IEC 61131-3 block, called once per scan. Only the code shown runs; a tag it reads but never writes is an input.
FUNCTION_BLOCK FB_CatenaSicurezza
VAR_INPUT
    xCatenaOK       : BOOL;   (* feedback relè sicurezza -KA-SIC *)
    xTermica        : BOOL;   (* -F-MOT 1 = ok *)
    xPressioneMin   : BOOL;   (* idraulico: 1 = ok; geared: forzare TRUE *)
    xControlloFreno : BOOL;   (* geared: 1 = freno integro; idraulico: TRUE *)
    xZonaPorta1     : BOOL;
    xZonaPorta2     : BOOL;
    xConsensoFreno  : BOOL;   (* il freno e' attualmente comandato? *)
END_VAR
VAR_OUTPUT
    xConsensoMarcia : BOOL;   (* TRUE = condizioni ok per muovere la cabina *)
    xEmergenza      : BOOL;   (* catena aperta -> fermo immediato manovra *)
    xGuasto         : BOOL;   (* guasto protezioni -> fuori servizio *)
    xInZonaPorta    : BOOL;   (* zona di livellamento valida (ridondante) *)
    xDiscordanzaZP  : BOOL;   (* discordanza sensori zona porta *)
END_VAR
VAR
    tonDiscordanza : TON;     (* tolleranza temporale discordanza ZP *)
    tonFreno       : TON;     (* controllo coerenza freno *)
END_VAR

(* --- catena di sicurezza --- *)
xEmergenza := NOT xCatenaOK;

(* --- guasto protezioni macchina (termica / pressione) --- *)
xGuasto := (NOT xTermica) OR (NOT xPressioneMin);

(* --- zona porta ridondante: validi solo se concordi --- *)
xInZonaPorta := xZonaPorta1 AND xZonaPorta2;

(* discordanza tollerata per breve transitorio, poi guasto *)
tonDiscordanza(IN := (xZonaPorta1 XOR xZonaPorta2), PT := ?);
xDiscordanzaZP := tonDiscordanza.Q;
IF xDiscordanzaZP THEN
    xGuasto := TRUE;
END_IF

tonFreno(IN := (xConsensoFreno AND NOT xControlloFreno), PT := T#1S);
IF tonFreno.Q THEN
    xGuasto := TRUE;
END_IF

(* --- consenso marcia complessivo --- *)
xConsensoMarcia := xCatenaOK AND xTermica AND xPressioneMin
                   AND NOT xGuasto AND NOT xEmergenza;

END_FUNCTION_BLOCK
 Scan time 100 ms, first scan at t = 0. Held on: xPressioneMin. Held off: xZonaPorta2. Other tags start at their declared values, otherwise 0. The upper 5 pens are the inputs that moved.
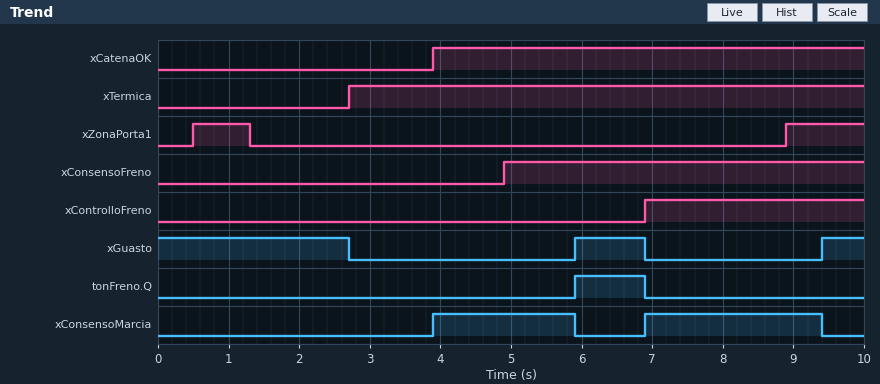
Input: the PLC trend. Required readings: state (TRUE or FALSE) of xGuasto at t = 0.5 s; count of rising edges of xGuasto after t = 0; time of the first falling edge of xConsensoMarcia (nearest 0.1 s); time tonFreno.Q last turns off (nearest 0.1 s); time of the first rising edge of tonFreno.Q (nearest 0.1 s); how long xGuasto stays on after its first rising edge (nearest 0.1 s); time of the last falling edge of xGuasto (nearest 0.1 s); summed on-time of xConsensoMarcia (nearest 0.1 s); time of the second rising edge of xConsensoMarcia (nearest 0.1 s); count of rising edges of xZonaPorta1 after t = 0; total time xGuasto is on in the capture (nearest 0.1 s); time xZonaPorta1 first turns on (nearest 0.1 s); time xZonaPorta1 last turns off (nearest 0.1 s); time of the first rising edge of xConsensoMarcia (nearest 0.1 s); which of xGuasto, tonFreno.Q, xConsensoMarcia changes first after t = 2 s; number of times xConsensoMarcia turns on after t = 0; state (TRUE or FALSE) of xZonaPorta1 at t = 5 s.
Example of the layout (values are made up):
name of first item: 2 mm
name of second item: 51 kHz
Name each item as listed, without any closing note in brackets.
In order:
state (TRUE or FALSE) of xGuasto at t = 0.5 s: TRUE
count of rising edges of xGuasto after t = 0: 2
time of the first falling edge of xConsensoMarcia: 5.9 s
time tonFreno.Q last turns off: 6.9 s
time of the first rising edge of tonFreno.Q: 5.9 s
how long xGuasto stays on after its first rising edge: 1.0 s
time of the last falling edge of xGuasto: 6.9 s
summed on-time of xConsensoMarcia: 4.5 s
time of the second rising edge of xConsensoMarcia: 6.9 s
count of rising edges of xZonaPorta1 after t = 0: 2
total time xGuasto is on in the capture: 4.3 s
time xZonaPorta1 first turns on: 0.5 s
time xZonaPorta1 last turns off: 1.3 s
time of the first rising edge of xConsensoMarcia: 3.9 s
which of xGuasto, tonFreno.Q, xConsensoMarcia changes first after t = 2 s: xGuasto
number of times xConsensoMarcia turns on after t = 0: 2
state (TRUE or FALSE) of xZonaPorta1 at t = 5 s: FALSE
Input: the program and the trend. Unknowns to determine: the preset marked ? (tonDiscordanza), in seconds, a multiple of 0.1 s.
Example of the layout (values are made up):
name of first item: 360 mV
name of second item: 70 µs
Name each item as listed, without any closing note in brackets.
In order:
the preset marked ? (tonDiscordanza), in seconds, a multiple of 0.1 s: 0.5 s
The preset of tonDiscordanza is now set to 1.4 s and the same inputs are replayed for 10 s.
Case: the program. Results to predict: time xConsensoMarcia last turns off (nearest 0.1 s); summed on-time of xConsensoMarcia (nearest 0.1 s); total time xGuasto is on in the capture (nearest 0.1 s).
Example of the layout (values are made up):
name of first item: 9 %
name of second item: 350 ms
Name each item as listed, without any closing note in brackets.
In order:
time xConsensoMarcia last turns off: 5.9 s
summed on-time of xConsensoMarcia: 5.1 s
total time xGuasto is on in the capture: 3.7 s
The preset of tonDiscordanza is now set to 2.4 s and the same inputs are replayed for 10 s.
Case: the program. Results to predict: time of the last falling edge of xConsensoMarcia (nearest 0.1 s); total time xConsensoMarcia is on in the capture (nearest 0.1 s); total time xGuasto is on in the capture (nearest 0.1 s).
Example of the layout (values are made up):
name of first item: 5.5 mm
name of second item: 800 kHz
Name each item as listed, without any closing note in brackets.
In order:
time of the last falling edge of xConsensoMarcia: 5.9 s
total time xConsensoMarcia is on in the capture: 5.1 s
total time xGuasto is on in the capture: 3.7 s
